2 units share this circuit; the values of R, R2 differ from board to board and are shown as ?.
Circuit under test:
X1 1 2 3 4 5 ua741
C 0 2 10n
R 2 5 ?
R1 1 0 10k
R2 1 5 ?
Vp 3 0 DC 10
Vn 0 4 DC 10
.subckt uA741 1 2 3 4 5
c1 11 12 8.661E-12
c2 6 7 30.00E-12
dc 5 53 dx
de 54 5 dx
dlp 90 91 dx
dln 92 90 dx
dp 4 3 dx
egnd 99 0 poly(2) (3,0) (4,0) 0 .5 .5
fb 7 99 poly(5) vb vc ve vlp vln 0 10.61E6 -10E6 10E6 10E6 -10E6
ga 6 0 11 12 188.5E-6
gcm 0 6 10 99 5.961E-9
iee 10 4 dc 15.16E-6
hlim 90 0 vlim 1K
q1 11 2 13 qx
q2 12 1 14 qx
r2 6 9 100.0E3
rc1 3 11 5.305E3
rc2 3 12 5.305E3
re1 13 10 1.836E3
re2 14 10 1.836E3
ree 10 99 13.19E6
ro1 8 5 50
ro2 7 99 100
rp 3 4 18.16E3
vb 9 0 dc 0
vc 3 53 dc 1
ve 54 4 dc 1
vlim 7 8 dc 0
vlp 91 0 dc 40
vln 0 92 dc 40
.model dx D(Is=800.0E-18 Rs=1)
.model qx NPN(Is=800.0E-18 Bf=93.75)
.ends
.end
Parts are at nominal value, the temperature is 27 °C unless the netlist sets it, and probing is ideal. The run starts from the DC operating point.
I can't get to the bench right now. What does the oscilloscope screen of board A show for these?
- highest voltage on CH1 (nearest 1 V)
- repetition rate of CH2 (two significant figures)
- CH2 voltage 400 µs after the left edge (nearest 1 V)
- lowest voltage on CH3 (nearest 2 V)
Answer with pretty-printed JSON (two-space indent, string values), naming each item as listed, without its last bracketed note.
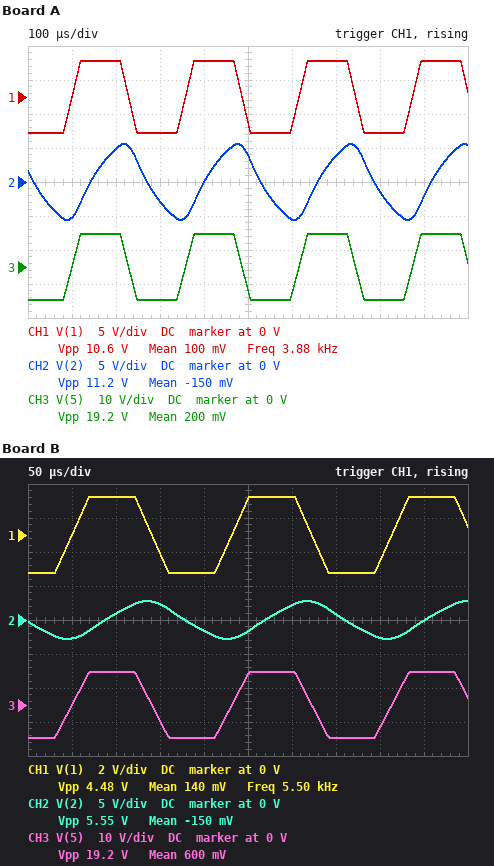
{
  "highest voltage on CH1": "5 V",
  "repetition rate of CH2": "3.9 kHz",
  "CH2 voltage 400 µs after the left edge": "0 V",
  "lowest voltage on CH3": "-10 V"
}
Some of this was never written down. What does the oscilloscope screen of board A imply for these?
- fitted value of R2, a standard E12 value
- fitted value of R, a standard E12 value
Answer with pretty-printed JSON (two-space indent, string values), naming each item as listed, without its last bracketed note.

{
  "fitted value of R2, a standard E12 value": "8.2 kΩ",
  "fitted value of R, a standard E12 value": "8.2 kΩ"
}
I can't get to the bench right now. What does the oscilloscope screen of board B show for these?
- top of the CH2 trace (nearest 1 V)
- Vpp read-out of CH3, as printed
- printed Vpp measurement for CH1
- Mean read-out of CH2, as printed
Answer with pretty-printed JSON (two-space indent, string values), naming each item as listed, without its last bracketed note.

{
  "top of the CH2 trace": "3 V",
  "Vpp read-out of CH3, as printed": "19.2 V",
  "printed Vpp measurement for CH1": "4.48 V",
  "Mean read-out of CH2, as printed": "-150 mV"
}
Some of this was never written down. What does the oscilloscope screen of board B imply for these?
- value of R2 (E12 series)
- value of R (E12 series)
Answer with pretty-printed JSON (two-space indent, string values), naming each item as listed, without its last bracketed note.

{
  "value of R2": "33 kΩ",
  "value of R": "12 kΩ"
}
